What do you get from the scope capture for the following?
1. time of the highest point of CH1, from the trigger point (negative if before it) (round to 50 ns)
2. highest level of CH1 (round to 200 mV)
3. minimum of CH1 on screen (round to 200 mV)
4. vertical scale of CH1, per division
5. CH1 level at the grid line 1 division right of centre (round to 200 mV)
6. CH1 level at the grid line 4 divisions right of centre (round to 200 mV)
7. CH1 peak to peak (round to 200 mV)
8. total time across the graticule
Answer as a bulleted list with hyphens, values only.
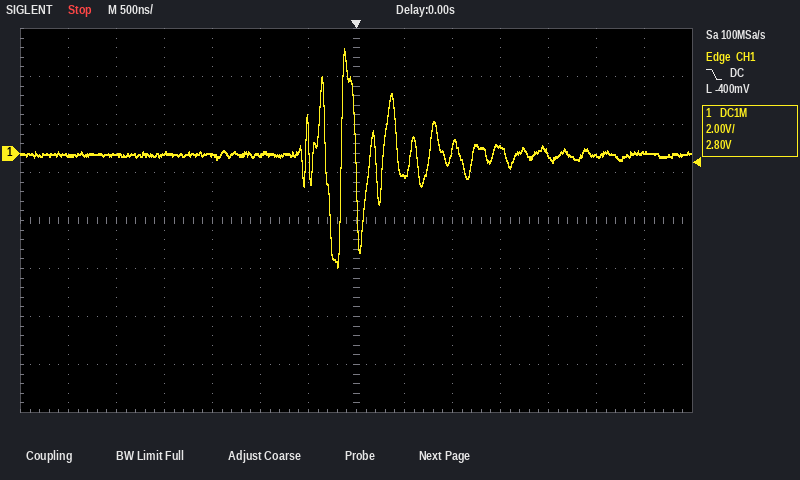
- -100 ns
- 4.4 V
- -4.8 V
- 2 V
- -1.0 V
- 0.0 V
- 9.2 V
- 7 µs
